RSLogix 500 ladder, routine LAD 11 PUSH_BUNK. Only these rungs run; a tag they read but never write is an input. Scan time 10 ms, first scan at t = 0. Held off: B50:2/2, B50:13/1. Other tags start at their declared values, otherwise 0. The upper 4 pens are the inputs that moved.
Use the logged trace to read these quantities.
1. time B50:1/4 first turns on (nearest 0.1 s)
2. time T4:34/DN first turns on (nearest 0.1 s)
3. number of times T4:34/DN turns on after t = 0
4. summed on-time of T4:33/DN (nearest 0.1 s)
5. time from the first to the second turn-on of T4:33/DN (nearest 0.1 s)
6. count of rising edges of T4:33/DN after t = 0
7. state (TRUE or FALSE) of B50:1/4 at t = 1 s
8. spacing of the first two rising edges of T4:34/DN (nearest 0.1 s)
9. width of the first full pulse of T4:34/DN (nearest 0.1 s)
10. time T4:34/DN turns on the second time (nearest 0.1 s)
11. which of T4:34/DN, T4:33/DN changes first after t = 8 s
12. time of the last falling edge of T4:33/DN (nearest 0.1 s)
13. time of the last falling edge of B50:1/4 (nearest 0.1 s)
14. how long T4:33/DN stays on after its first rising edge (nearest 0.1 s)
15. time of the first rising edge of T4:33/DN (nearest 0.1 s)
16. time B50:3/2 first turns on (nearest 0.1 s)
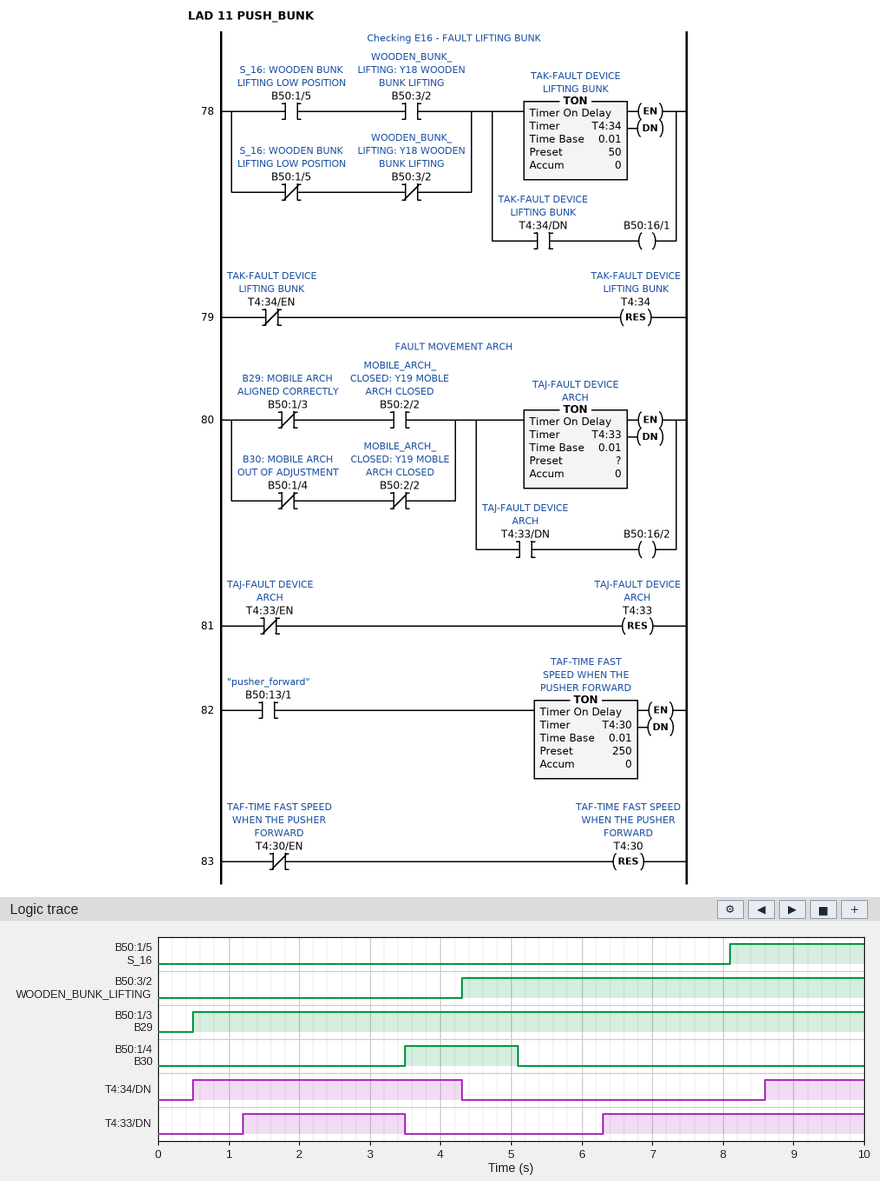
3.5 s
0.5 s
2
6.0 s
5.1 s
2
FALSE
8.1 s
3.8 s
8.6 s
T4:34/DN
3.5 s
5.1 s
2.3 s
1.2 s
4.3 s
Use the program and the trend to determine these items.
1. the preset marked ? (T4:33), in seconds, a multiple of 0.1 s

1.2 s
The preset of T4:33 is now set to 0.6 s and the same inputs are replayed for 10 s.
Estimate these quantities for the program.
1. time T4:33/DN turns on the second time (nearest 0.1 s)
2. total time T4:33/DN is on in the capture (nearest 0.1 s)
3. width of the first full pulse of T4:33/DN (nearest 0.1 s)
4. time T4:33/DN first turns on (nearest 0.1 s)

5.7 s
7.2 s
2.9 s
0.6 s
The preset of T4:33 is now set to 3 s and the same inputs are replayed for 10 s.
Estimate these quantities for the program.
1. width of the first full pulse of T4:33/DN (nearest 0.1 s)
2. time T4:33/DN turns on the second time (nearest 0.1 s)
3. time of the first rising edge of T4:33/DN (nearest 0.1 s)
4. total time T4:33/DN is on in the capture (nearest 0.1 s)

0.5 s
8.1 s
3.0 s
2.4 s
